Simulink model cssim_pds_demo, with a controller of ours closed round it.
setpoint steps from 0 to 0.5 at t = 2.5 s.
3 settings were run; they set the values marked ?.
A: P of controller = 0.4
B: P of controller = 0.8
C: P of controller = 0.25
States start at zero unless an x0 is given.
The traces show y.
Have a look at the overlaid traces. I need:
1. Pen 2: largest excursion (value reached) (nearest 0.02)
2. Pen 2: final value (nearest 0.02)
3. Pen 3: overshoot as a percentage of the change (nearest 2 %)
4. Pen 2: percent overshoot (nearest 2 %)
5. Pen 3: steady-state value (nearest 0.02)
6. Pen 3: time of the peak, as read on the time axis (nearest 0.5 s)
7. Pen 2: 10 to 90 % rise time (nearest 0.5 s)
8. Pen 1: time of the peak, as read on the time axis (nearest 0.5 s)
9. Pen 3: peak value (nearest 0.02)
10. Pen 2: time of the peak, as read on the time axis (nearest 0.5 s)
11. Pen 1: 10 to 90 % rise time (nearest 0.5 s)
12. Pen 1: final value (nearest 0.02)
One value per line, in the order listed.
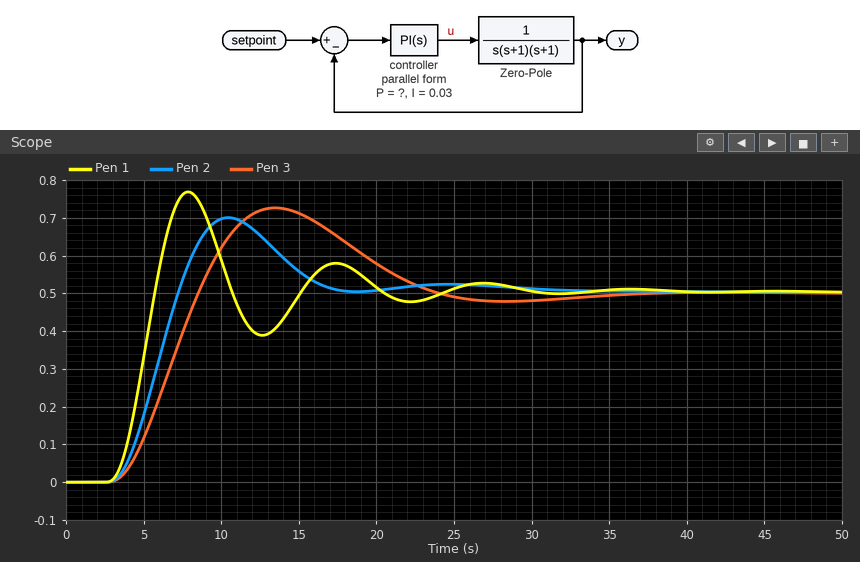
0.70
0.50
46 %
40 %
0.50
13.5 s
3.0 s
8.0 s
0.72
10.5 s
2.0 s
0.50
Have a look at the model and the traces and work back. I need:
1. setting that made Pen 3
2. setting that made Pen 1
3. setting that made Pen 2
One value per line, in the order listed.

C
B
A
